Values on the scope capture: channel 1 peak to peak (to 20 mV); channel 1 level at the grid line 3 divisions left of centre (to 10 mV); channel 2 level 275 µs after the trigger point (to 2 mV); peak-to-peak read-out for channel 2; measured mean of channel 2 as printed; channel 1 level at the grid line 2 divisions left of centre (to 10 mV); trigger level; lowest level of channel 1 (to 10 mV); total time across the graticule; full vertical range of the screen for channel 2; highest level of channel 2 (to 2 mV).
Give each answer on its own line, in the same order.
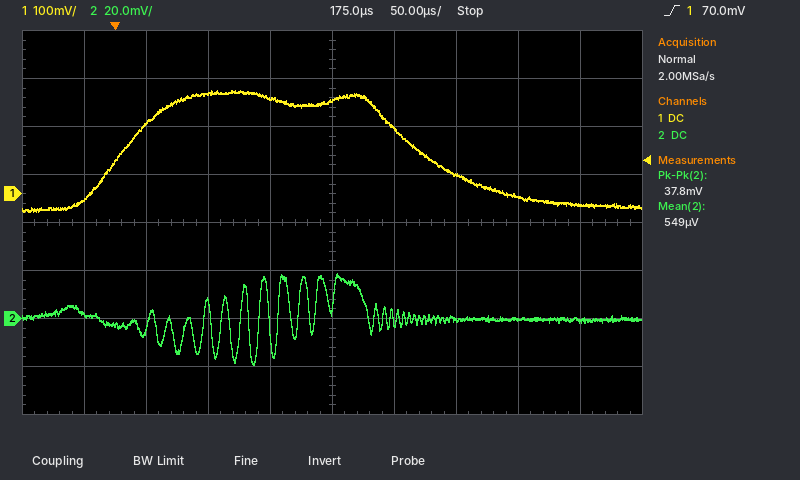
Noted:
260 mV
150 mV
0 mV
37.8 mV
549 µV
210 mV
70.0 mV
-40 mV
500 µs
160 mV
18 mV
